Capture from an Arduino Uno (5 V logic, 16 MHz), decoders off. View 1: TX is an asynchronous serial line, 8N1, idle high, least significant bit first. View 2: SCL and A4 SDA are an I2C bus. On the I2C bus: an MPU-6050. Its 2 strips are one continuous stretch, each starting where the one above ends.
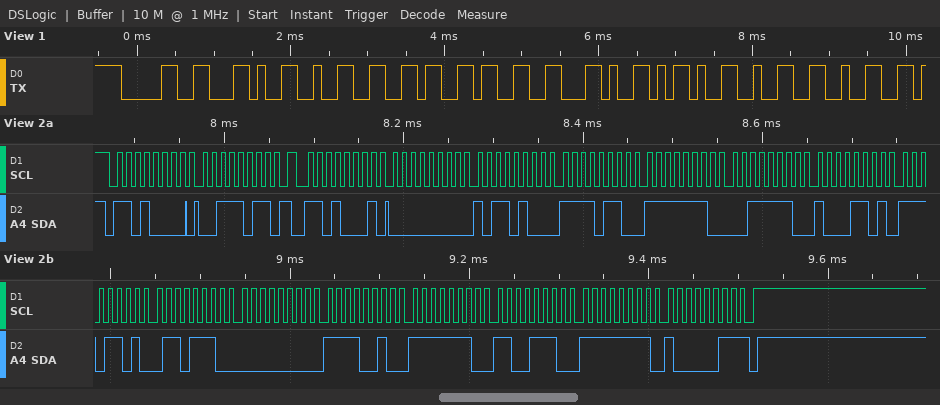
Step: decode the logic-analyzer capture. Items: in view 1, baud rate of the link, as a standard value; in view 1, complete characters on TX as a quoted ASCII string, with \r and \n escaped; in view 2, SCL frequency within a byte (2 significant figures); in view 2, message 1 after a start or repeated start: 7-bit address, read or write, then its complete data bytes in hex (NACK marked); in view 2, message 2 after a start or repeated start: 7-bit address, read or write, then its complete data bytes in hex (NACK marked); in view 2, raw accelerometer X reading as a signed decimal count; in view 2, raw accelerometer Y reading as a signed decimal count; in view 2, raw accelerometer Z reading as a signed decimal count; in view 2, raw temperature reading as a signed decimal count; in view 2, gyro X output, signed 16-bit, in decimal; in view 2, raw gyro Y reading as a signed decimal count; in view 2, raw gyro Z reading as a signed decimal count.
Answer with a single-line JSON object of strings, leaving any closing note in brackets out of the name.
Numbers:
{"in view 1, baud rate of the link, as a standard value": "9600 baud", "in view 1, complete characters on TX as a quoted ASCII string, with \\r and \\n escaped": "\"0,263,-22\"", "in view 2, SCL frequency within a byte": "100 kHz", "in view 2, message 1 after a start or repeated start: 7-bit address, read or write, then its complete data bytes in hex": "0x68 write: 3B", "in view 2, message 2 after a start or repeated start: 7-bit address, read or write, then its complete data bytes in hex": "0x68 read: 00 B4 F6 FE 3E 8D ED 6E 00 F2 FE CE FF 83 NACK", "in view 2, raw accelerometer X reading as a signed decimal count": "180", "in view 2, raw accelerometer Y reading as a signed decimal count": "-2306", "in view 2, raw accelerometer Z reading as a signed decimal count": "16013", "in view 2, raw temperature reading as a signed decimal count": "-4754", "in view 2, gyro X output, signed 16-bit, in decimal": "242", "in view 2, raw gyro Y reading as a signed decimal count": "-306", "in view 2, raw gyro Z reading as a signed decimal count": "-125"}
